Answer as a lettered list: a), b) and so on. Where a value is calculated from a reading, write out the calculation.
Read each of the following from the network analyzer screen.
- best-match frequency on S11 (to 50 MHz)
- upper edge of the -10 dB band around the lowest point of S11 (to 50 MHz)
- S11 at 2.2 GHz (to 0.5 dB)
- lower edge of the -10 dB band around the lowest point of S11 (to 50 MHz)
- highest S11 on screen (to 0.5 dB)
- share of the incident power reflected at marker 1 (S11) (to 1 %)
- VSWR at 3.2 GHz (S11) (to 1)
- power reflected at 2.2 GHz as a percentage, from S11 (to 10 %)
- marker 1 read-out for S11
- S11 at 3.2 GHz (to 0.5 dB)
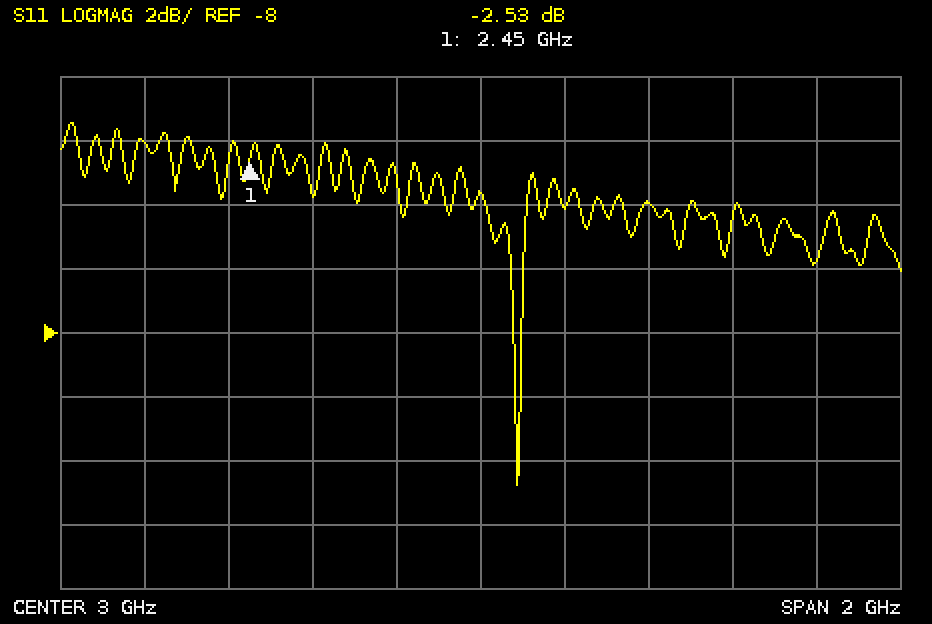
a) 3.10 GHz
b) 3.10 GHz
c) -2.0 dB
d) 3.10 GHz
e) -1.5 dB
f) 10^(-2.53/10) ≈ 56 %
g) |Γ| = 10^(-4/20) = 0.6310; VSWR = (1 + 0.6310)/(1 − 0.6310) ≈ 4
h) 10^(-2/10) ≈ 63.1 %, so 60 % to the nearest 10 %
i) -2.53 dB
j) -4.0 dB
